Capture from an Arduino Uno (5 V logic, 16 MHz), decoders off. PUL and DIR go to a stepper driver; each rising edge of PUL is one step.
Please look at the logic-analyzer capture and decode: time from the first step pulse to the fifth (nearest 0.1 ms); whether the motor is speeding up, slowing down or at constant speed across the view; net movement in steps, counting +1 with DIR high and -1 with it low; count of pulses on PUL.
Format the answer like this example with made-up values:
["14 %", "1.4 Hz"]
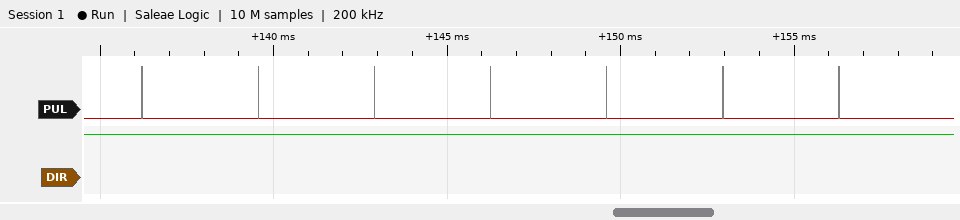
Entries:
["13.4 ms", "constant speed", "+7", "7"]
